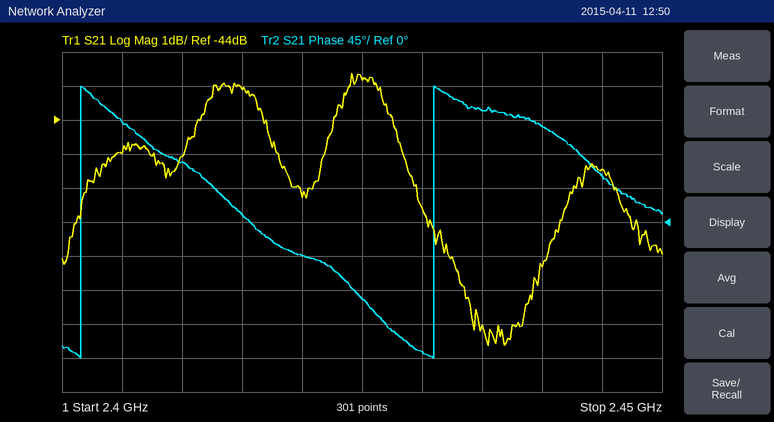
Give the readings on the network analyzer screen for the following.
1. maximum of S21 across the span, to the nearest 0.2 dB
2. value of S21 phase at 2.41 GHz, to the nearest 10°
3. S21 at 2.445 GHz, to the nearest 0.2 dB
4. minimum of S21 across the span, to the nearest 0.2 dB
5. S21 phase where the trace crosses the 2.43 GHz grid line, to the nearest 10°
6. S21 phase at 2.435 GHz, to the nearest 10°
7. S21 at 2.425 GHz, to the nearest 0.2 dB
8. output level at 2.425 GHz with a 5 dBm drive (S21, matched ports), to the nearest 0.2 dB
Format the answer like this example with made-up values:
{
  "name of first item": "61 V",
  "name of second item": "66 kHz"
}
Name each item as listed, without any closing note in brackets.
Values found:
{
  "maximum of S21 across the span, to the nearest 0.2 dB": "-42.6 dB",
  "value of S21 phase at 2.41 GHz, to the nearest 10°": "80°",
  "S21 at 2.445 GHz, to the nearest 0.2 dB": "-45.4 dB",
  "minimum of S21 across the span, to the nearest 0.2 dB": "-50.6 dB",
  "S21 phase where the trace crosses the 2.43 GHz grid line, to the nearest 10°": "-170°",
  "S21 phase at 2.435 GHz, to the nearest 10°": "150°",
  "S21 at 2.425 GHz, to the nearest 0.2 dB": "-42.8 dB",
  "output level at 2.425 GHz with a 5 dBm drive (S21, matched ports), to the nearest 0.2 dB": "-37.8 dBm"
}
